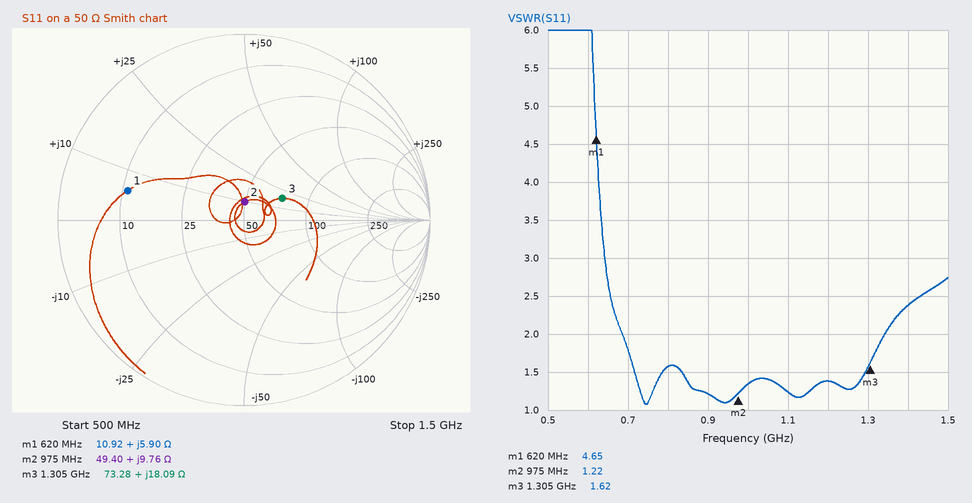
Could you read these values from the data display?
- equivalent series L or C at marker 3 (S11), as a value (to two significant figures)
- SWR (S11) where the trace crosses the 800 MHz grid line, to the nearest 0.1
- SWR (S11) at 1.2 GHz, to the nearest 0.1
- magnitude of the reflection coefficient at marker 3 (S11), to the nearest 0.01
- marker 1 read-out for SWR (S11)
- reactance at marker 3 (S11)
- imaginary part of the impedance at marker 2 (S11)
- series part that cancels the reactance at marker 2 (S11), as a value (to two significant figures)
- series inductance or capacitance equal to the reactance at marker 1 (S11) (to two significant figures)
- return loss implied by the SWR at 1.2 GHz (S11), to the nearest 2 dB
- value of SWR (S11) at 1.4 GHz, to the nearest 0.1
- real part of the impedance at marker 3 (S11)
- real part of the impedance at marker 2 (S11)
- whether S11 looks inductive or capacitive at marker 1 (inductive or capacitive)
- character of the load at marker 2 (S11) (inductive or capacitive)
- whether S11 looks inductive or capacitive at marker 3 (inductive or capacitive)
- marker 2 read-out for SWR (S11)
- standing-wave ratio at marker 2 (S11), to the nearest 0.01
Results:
2.2 nH
1.6
1.4
0.24
4.65
+18.09 Ω
+9.76 Ω
17 pF
1.5 nH
16 dB
2.4
73.28 Ω
49.40 Ω
inductive
inductive
inductive
1.22
1.22
